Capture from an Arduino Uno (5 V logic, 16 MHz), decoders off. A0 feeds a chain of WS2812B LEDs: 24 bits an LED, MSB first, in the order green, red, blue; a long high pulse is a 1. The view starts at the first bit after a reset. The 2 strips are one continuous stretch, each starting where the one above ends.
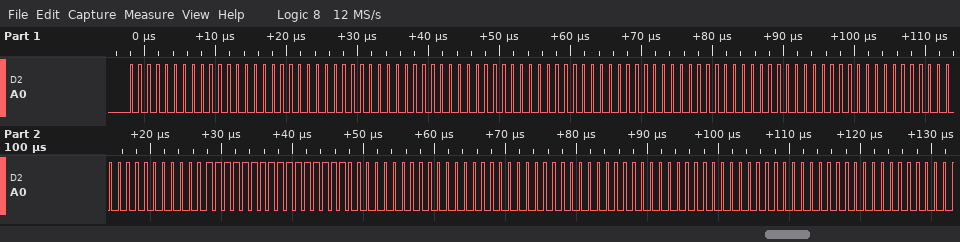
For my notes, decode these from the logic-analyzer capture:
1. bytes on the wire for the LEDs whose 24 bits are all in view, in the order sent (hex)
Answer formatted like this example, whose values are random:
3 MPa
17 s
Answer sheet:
00 00 00 00 00 00 00 00 00 00 00 00 00 FF FF 00 00 00 00 00 00
